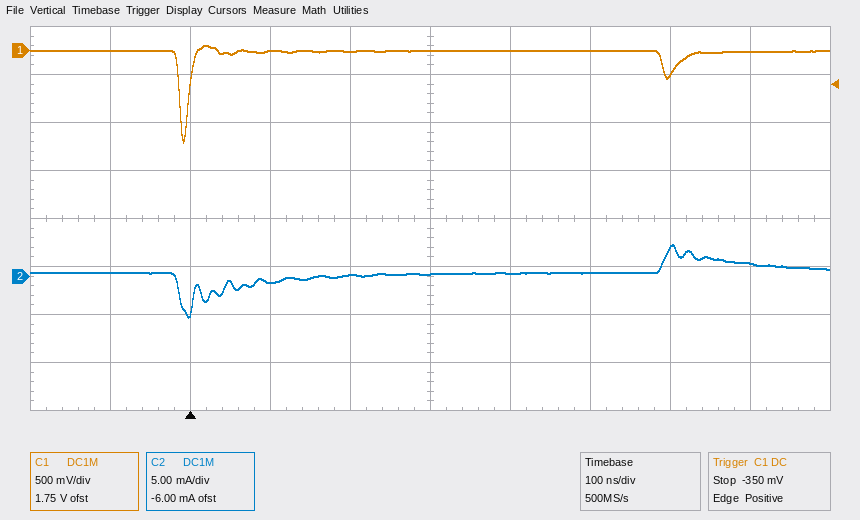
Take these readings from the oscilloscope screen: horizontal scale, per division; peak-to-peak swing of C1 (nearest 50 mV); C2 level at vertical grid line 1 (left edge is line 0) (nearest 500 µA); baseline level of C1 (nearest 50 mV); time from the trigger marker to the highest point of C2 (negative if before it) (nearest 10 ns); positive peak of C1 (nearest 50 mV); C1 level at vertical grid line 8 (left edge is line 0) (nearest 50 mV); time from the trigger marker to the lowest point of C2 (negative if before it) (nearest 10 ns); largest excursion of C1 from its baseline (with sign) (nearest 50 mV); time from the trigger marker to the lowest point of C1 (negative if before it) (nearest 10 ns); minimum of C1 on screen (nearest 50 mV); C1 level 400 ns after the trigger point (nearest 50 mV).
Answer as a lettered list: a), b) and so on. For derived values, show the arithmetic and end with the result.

a) 100 ns
b) 50 mV − (-950 mV) = 1.00 V
c) 500 µA
d) 0 mV
e) +600 ns
f) 50 mV
g) -250 mV
h) 0 ns
i) -950 mV − (0 mV) = -950 mV
j) -10 ns
k) -950 mV
l) 0 mV
